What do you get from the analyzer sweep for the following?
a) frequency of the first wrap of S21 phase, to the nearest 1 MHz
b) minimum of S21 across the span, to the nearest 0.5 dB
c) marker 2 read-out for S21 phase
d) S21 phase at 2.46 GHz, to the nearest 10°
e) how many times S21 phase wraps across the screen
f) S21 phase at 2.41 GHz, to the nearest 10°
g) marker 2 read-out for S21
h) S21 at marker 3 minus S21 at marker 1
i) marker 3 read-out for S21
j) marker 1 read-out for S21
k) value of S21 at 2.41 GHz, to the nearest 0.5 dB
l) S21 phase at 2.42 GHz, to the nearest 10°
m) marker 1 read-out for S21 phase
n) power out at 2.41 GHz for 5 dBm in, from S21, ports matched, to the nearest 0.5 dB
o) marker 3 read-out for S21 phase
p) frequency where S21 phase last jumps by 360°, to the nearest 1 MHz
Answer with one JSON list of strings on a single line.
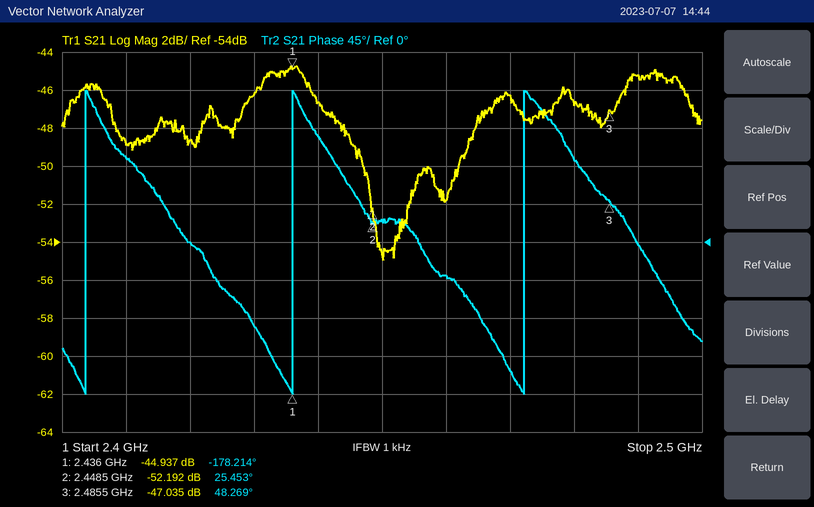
["2.404 GHz", "-55.0 dB", "25.453°", "-40°", "3", "100°", "-52.192 dB", "-2.098 dB", "-47.035 dB", "-44.937 dB", "-49.0 dB", "0°", "-178.214°", "-44.0 dBm", "48.269°", "2.472 GHz"]
